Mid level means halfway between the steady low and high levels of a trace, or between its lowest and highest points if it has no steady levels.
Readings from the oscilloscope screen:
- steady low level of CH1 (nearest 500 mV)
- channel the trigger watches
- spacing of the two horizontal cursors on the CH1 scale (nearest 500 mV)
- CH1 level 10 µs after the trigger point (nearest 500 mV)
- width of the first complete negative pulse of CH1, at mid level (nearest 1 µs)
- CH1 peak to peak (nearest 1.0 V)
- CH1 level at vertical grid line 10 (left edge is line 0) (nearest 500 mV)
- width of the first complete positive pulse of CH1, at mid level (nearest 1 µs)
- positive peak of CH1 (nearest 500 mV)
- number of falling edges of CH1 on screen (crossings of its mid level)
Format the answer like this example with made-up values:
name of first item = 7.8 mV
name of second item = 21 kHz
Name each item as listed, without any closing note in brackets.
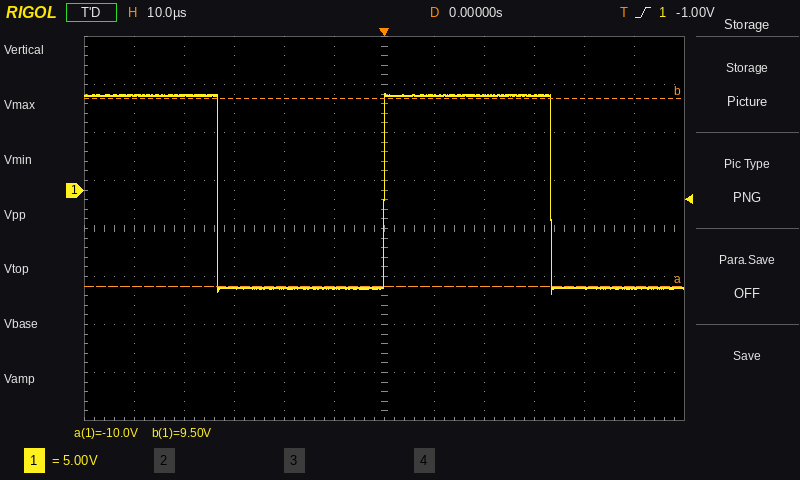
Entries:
steady low level of CH1 = -10.0 V
channel the trigger watches = CH1
spacing of the two horizontal cursors on the CH1 scale = 19.5 V
CH1 level 10 µs after the trigger point = 10.0 V
width of the first complete negative pulse of CH1, at mid level = 33 µs
CH1 peak to peak = 21.0 V
CH1 level at vertical grid line 10 (left edge is line 0) = -10.0 V
width of the first complete positive pulse of CH1, at mid level = 33 µs
positive peak of CH1 = 10.0 V
number of falling edges of CH1 on screen = 2
